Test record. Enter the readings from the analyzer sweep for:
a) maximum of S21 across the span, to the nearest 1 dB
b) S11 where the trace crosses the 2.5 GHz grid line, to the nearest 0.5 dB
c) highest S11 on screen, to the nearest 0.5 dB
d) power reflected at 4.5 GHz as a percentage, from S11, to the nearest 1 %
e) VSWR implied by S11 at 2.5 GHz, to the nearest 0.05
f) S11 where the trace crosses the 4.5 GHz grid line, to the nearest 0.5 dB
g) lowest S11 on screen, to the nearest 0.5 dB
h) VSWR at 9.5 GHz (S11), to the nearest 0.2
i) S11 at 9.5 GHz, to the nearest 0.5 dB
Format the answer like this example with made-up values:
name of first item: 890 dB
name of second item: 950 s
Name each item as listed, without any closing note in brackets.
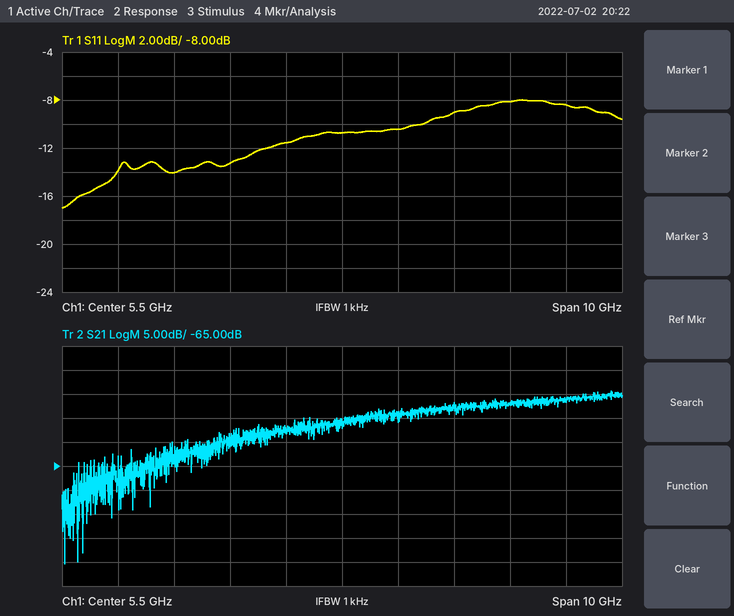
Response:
maximum of S21 across the span, to the nearest 1 dB: -49 dB
S11 where the trace crosses the 2.5 GHz grid line, to the nearest 0.5 dB: -14.0 dB
highest S11 on screen, to the nearest 0.5 dB: -8.0 dB
power reflected at 4.5 GHz as a percentage, from S11, to the nearest 1 %: 7 %
VSWR implied by S11 at 2.5 GHz, to the nearest 0.05: 1.50
S11 where the trace crosses the 4.5 GHz grid line, to the nearest 0.5 dB: -11.5 dB
lowest S11 on screen, to the nearest 0.5 dB: -17.0 dB
VSWR at 9.5 GHz (S11), to the nearest 0.2: 2.2
S11 at 9.5 GHz, to the nearest 0.5 dB: -8.5 dB
